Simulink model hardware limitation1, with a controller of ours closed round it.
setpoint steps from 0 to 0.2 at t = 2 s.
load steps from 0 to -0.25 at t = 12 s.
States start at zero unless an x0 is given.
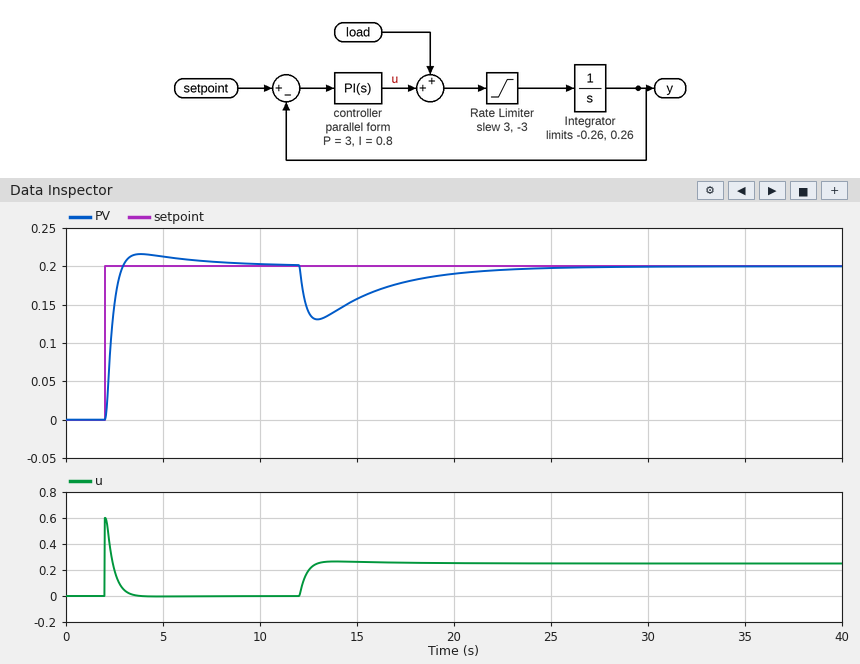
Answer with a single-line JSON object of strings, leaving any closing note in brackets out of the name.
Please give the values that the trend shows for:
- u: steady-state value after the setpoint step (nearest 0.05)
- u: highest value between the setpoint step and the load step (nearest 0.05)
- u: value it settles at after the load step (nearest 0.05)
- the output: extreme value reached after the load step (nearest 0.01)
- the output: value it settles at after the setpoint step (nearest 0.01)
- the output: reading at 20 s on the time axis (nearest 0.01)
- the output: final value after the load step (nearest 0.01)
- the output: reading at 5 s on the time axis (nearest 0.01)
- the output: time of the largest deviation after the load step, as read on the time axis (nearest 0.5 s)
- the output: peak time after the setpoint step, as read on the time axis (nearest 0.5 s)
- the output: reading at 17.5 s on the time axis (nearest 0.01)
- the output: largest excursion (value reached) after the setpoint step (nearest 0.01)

{"u: steady-state value after the setpoint step": "0.00", "u: highest value between the setpoint step and the load step": "0.60", "u: value it settles at after the load step": "0.25", "the output: extreme value reached after the load step": "0.13", "the output: value it settles at after the setpoint step": "0.20", "the output: reading at 20 s on the time axis": "0.19", "the output: final value after the load step": "0.20", "the output: reading at 5 s on the time axis": "0.21", "the output: time of the largest deviation after the load step, as read on the time axis": "13.0 s", "the output: peak time after the setpoint step, as read on the time axis": "4.0 s", "the output: reading at 17.5 s on the time axis": "0.18", "the output: largest excursion (value reached) after the setpoint step": "0.22"}
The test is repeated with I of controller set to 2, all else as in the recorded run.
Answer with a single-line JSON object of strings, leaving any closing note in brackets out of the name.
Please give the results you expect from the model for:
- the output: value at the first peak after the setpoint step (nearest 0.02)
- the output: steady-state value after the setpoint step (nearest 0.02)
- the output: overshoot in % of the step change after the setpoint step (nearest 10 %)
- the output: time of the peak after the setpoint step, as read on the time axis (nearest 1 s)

{"the output: value at the first peak after the setpoint step": "0.24", "the output: steady-state value after the setpoint step": "0.20", "the output: overshoot in % of the step change after the setpoint step": "20 %", "the output: time of the peak after the setpoint step, as read on the time axis": "3 s"}
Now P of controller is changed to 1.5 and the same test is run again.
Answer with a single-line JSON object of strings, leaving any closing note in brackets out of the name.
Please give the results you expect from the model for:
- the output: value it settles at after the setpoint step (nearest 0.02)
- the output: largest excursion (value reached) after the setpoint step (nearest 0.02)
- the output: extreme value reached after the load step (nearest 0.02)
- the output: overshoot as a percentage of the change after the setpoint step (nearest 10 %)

{"the output: value it settles at after the setpoint step": "0.20", "the output: largest excursion (value reached) after the setpoint step": "0.24", "the output: extreme value reached after the load step": "0.08", "the output: overshoot as a percentage of the change after the setpoint step": "20 %"}
